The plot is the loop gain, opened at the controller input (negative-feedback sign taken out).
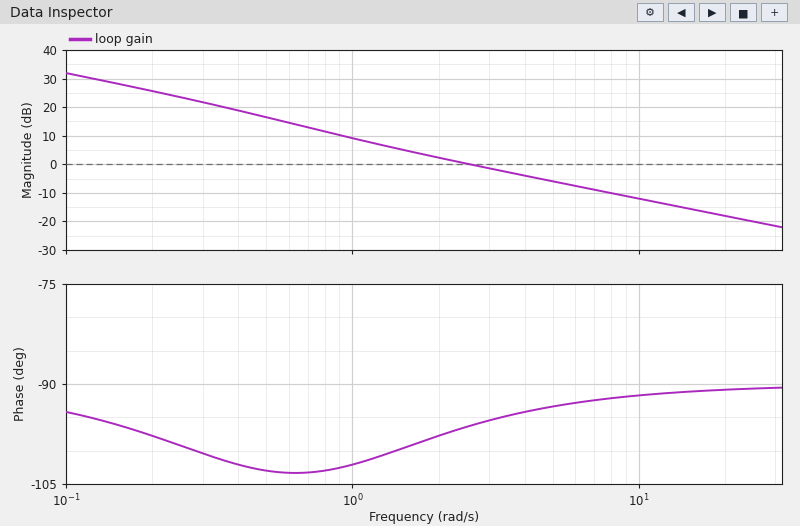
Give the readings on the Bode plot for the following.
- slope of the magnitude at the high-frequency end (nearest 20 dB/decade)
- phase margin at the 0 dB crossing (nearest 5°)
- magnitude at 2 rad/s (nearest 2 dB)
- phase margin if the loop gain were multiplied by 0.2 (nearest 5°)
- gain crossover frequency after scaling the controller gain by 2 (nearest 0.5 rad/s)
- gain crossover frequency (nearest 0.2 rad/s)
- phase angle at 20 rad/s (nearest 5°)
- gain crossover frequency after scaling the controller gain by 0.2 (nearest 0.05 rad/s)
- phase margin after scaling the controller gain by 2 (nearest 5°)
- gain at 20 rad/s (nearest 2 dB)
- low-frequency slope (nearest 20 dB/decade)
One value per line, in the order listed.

-20 dB/decade
85°
2 dB
75°
5.0 rad/s
2.6 rad/s
-90°
0.65 rad/s
85°
-18 dB
-20 dB/decade
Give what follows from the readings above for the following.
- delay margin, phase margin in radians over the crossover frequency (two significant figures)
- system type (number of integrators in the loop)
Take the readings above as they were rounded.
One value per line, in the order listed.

0.57 s
1
